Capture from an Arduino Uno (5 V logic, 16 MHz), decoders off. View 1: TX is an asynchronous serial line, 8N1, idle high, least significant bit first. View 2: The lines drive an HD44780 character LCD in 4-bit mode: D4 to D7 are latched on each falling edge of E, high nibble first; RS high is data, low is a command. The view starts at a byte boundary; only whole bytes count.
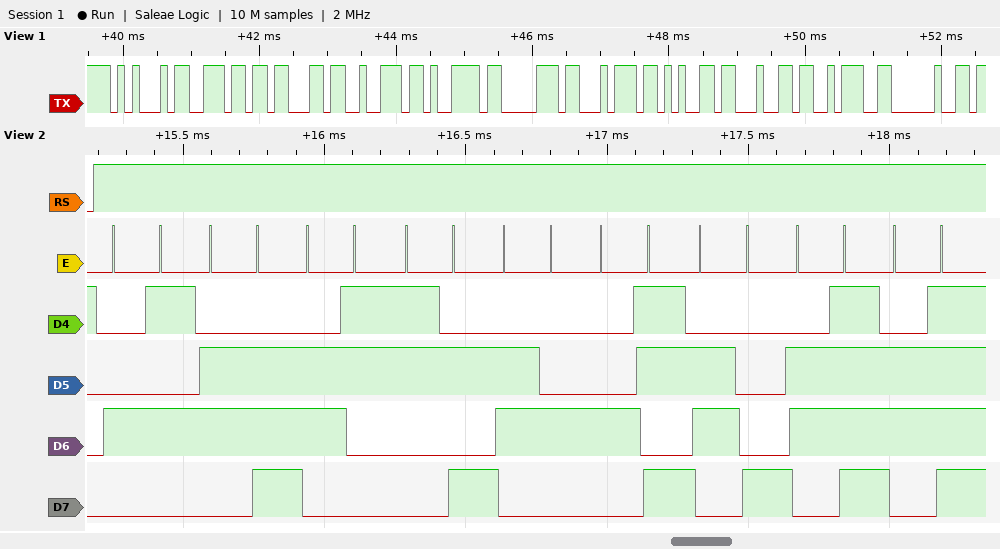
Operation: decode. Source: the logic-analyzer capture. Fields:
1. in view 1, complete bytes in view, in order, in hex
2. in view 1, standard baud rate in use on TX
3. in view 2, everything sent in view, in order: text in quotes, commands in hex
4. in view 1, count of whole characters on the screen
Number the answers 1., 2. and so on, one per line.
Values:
1. 45 6E 63 72 79 70 74 65 64 3A 20
2. 9600 baud
3. "Enc:dKhoo"
4. 11
